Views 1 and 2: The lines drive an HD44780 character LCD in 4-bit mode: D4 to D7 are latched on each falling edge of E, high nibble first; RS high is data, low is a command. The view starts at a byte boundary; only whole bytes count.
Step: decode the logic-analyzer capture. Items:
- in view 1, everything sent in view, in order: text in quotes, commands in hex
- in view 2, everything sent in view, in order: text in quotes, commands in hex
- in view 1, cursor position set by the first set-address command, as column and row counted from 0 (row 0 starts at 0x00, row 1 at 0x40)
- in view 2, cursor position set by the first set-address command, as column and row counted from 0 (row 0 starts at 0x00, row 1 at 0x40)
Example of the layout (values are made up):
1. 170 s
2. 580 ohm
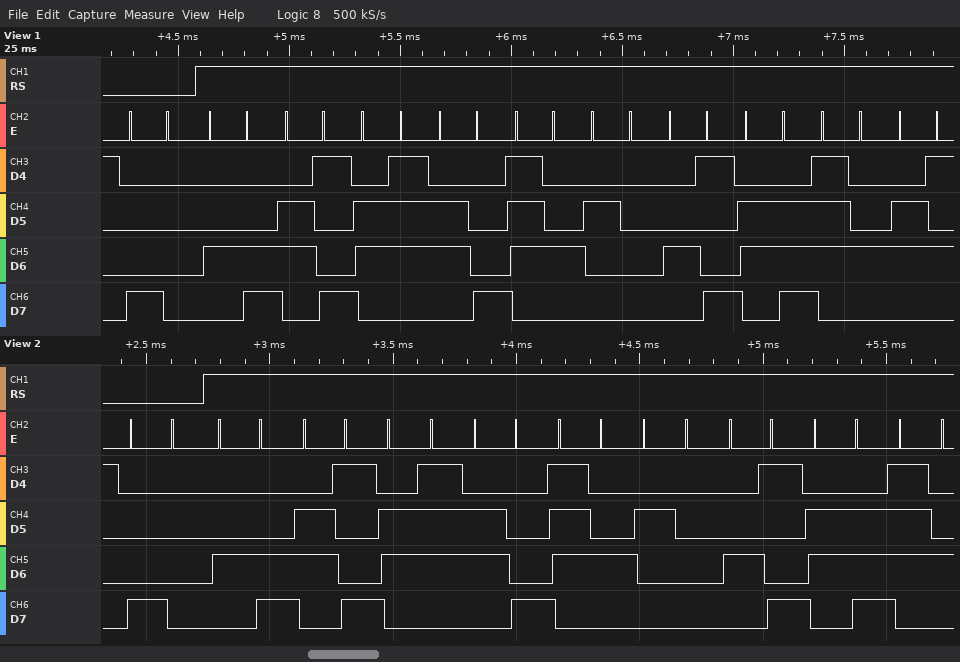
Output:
1. 0x80 "Light Inte"
2. 0x80 "Light Int"
3. column 0, row 0
4. column 0, row 0
